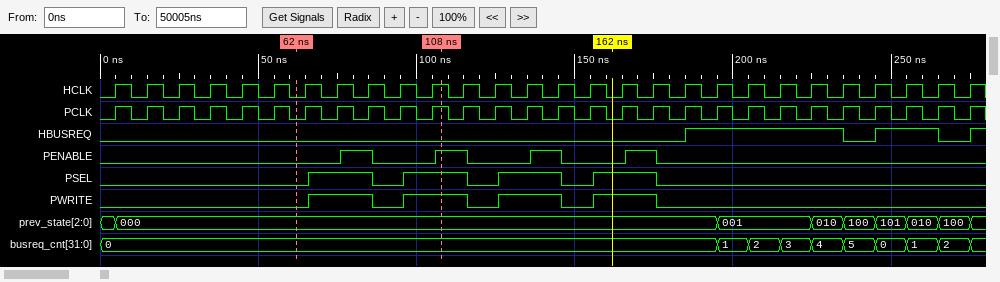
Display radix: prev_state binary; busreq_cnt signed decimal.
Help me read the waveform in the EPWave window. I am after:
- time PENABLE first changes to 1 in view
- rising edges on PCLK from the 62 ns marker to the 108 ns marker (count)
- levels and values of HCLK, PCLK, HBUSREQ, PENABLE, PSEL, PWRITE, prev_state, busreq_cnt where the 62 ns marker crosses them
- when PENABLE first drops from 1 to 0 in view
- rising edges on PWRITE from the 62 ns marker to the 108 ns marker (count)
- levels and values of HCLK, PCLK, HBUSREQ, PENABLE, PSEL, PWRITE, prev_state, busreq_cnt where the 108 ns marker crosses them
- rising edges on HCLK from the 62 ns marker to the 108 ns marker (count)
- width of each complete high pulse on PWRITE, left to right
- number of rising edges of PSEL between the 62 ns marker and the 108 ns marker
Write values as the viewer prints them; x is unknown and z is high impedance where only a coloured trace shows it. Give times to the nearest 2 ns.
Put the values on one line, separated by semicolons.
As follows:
76 ns; 5; HCLK=0, PCLK=0, HBUSREQ=0, PENABLE=0, PSEL=0, PWRITE=0, prev_state=000, busreq_cnt=0; 86 ns; 2; HCLK=1, PCLK=1, HBUSREQ=0, PENABLE=1, PSEL=1, PWRITE=1, prev_state=000, busreq_cnt=0; 5; 20 ns, 20 ns, 20 ns, 20 ns; 2
